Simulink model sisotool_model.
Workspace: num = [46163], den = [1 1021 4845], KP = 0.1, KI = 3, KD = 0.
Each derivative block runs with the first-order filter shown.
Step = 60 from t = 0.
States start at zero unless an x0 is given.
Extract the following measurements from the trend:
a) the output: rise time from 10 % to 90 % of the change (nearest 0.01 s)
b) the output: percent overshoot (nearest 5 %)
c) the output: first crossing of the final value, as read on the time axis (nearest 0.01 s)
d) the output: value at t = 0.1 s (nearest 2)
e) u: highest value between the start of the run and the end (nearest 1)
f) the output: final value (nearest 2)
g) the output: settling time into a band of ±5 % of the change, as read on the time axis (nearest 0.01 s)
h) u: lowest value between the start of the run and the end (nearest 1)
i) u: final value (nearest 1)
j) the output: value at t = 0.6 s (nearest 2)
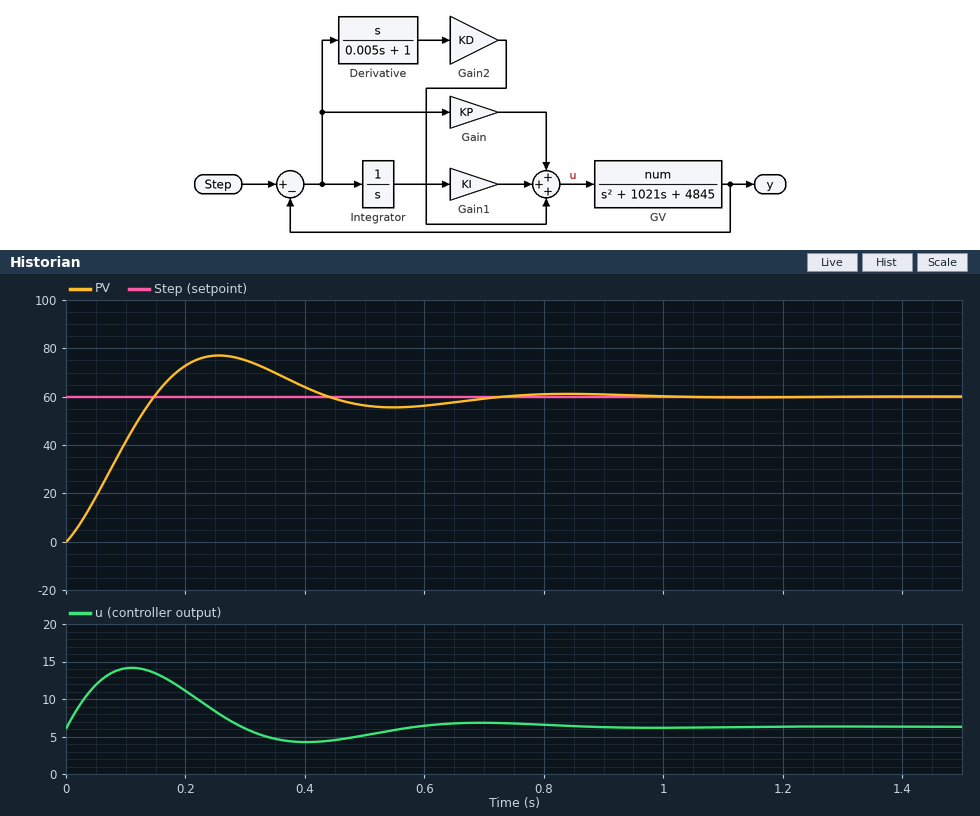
0.11 s
30 %
0.15 s
42
14
60
0.63 s
4
6
56
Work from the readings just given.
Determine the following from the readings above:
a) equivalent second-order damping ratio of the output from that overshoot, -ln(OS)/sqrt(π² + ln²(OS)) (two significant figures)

0.36
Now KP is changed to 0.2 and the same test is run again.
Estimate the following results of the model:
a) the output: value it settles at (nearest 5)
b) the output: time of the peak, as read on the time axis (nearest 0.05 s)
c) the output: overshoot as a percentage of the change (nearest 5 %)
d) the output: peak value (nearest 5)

60
0.25 s
15 %
70
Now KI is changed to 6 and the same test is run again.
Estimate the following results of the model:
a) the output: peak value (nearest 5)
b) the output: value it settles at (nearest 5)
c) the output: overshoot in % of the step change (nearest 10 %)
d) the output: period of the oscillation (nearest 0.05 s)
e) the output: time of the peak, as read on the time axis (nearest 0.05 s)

85
60
40 %
0.40 s
0.20 s
